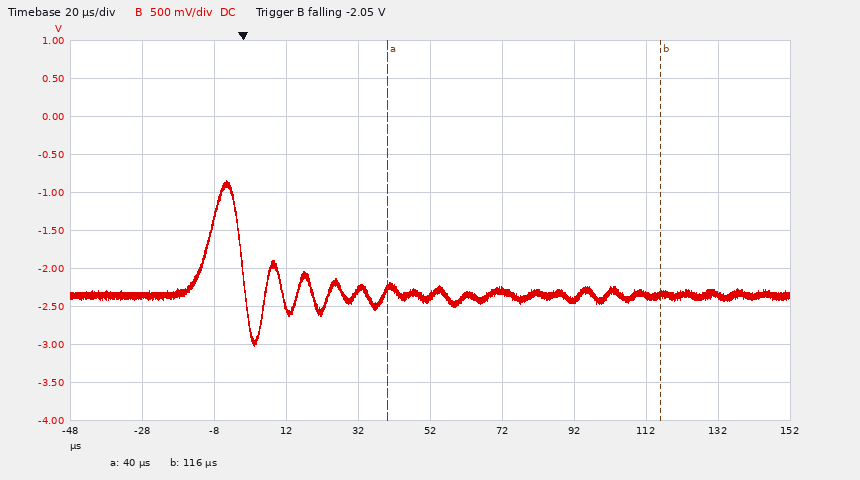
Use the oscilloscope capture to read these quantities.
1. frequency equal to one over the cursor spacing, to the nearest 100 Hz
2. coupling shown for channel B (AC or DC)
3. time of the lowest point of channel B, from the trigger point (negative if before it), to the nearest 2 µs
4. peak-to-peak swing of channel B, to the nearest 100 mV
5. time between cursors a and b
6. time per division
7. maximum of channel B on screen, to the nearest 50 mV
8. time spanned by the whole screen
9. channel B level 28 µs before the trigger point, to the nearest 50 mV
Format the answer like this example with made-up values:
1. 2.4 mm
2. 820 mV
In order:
1. 13.2 kHz
2. DC
3. +4 µs
4. 2.20 V
5. 76 µs
6. 20 µs
7. -850 mV
8. 200 µs
9. -2.35 V
